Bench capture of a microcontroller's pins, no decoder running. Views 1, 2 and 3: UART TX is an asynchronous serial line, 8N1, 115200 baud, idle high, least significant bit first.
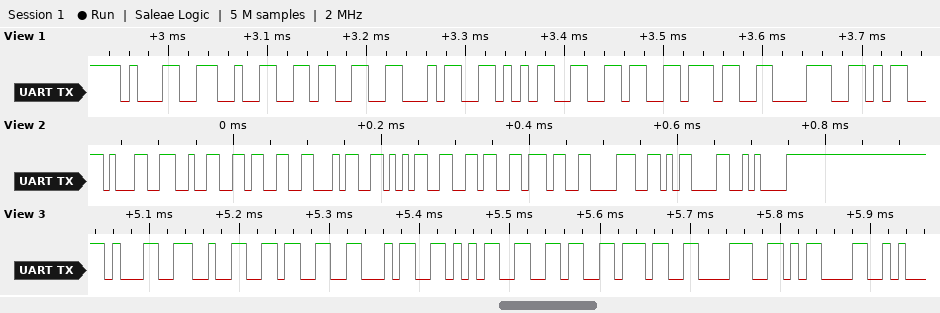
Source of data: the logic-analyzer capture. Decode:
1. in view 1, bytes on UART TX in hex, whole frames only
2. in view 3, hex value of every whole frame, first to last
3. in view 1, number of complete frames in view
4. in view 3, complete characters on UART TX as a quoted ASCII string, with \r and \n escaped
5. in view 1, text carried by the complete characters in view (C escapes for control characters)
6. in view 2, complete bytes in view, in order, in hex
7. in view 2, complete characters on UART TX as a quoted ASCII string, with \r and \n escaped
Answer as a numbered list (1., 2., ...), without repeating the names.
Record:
1. 31 32 33 34 35 36 37 38
2. 31 32 33 34 35 36 37 38 0D
3. 8
4. "12345678\r"
5. "12345678"
6. 31 32 33 34 35 36 37 38 0D 0A
7. "12345678\r\n"
